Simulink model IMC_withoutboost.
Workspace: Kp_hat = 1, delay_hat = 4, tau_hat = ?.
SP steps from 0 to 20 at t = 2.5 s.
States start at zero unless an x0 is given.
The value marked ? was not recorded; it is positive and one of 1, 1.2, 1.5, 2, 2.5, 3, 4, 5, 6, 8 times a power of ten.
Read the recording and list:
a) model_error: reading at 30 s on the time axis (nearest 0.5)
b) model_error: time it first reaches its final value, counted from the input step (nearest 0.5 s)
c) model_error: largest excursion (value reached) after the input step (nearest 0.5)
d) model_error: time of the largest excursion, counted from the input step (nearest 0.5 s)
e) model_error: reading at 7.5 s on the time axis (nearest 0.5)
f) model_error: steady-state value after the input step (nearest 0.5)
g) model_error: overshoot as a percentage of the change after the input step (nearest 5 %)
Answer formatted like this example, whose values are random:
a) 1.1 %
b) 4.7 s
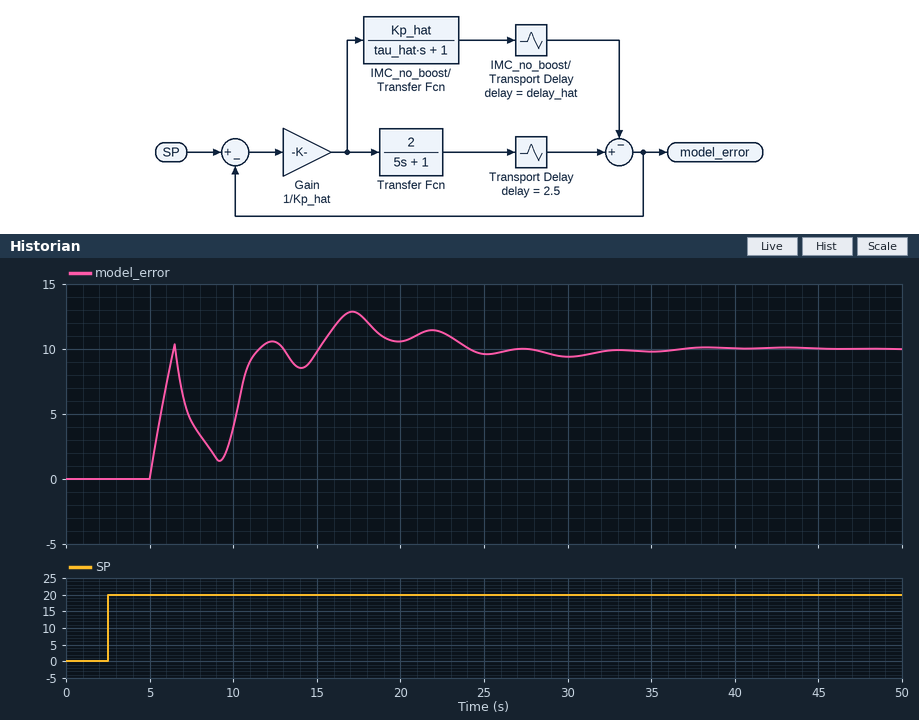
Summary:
a) 9.5
b) 4.0 s
c) 13.0
d) 14.5 s
e) 4.5
f) 10.0
g) 30 %
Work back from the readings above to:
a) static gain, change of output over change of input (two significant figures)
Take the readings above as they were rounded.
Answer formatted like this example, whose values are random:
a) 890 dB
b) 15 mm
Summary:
a) 0.50
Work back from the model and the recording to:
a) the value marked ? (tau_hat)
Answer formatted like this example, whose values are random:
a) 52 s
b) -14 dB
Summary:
a) 1.2
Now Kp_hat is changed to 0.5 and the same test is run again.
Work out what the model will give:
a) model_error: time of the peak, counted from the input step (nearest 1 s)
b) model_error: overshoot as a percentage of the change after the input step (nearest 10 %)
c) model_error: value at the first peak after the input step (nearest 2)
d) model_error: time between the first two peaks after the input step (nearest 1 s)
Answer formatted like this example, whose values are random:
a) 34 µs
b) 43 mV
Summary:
a) 4 s
b) 40 %
c) 20
d) 6 s
